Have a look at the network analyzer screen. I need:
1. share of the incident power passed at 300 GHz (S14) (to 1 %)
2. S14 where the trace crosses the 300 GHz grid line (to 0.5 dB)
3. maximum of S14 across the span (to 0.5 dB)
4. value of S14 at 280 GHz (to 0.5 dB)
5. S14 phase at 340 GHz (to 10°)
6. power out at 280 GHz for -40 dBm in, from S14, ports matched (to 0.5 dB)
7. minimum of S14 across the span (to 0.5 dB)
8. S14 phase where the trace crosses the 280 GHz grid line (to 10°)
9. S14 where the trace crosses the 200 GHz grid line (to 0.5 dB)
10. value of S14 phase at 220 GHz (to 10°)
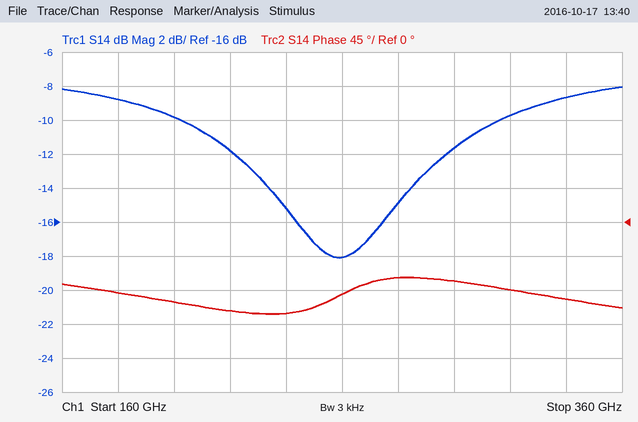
7 %
-11.5 dB
-8.0 dB
-15.0 dB
-100°
-55.0 dBm
-18.0 dB
-70°
-10.0 dB
-120°
